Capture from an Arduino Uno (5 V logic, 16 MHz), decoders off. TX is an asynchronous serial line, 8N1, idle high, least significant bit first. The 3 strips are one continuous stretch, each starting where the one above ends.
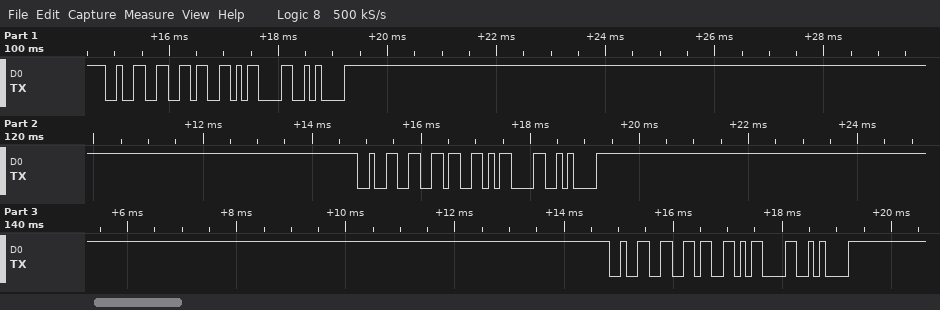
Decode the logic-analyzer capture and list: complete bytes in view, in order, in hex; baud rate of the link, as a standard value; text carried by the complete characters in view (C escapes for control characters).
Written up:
32 36 0D 0A 32 36 0D 0A 32 36 0D 0A
9600 baud
"26\r\n26\r\n26\r\n"
